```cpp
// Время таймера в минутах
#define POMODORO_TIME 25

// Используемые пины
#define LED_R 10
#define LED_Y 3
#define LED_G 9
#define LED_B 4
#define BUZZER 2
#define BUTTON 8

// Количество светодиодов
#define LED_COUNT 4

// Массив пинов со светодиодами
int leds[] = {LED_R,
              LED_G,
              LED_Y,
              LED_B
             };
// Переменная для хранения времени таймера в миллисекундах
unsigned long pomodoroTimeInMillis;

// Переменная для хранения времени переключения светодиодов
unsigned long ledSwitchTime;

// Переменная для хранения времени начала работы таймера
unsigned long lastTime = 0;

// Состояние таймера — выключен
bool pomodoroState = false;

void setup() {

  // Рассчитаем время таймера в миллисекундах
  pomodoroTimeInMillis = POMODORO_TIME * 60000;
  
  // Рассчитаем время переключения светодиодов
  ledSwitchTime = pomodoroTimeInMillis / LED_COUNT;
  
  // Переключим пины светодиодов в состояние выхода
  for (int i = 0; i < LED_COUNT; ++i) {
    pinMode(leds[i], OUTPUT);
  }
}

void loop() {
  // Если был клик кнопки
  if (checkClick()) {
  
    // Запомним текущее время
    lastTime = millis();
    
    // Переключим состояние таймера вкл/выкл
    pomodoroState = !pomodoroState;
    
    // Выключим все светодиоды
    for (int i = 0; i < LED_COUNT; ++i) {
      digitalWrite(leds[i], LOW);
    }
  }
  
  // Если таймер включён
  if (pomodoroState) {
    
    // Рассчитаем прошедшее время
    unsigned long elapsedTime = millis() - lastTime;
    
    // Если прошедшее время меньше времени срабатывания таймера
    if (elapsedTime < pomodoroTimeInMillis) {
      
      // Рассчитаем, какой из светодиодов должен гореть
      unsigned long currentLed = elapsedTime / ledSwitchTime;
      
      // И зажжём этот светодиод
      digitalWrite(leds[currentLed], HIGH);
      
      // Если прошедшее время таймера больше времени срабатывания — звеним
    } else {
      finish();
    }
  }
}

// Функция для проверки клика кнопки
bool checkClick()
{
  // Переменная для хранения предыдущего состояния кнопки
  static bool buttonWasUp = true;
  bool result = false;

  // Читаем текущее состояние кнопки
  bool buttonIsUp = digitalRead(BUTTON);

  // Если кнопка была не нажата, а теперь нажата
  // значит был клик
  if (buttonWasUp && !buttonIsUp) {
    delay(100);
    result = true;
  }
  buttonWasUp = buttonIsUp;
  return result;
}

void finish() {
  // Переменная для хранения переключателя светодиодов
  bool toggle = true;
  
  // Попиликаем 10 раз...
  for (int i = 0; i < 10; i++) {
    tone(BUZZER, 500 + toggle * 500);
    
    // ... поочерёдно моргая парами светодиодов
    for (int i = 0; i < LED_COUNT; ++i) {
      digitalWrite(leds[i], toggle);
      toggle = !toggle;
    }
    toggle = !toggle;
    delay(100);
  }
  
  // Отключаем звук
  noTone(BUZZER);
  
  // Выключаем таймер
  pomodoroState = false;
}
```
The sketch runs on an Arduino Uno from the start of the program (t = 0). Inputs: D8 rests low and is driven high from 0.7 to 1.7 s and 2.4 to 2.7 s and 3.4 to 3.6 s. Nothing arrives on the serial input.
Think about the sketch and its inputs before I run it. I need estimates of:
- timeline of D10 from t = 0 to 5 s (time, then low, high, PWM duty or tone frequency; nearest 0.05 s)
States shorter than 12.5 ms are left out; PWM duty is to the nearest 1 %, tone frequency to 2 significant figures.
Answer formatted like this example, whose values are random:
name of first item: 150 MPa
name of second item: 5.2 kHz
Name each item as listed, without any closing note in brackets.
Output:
timeline of D10 from t = 0 to 5 s: 0 s low; 0.1 s high; 1.8 s low; 2.8 s high; 3.7 s low
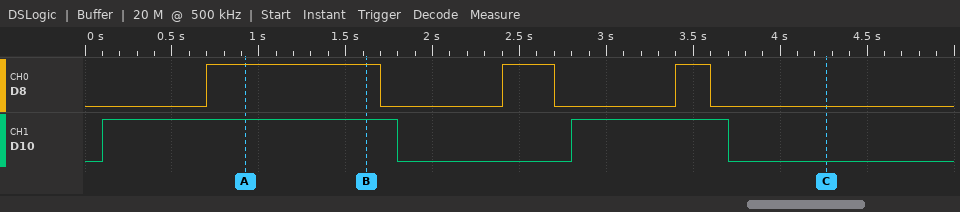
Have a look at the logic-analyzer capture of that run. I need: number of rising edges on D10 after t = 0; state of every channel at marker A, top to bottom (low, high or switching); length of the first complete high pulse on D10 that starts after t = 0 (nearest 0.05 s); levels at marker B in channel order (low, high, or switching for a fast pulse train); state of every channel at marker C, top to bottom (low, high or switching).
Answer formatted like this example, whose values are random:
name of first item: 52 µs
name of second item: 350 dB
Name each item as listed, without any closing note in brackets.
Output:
number of rising edges on D10 after t = 0: 2
state of every channel at marker A, top to bottom: D8 high, D10 high
length of the first complete high pulse on D10 that starts after t = 0: 1.70 s
levels at marker B in channel order: D8 high, D10 high
state of every channel at marker C, top to bottom: D8 low, D10 low
